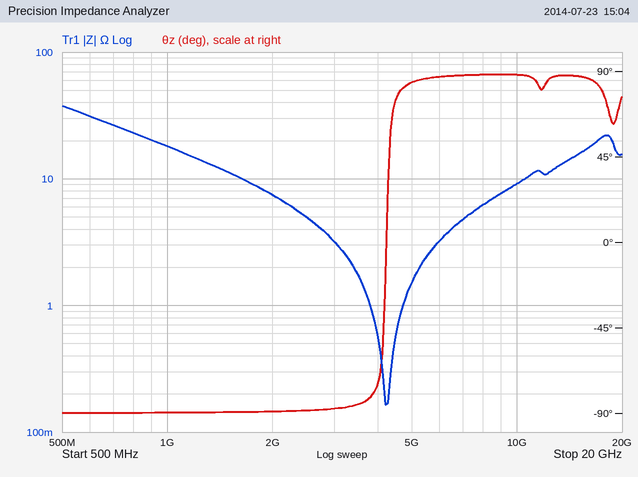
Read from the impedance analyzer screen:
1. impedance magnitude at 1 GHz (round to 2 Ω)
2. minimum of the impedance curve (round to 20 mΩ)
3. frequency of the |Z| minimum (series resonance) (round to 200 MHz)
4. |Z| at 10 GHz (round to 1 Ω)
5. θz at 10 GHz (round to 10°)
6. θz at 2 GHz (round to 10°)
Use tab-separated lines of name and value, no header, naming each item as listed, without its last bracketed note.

impedance magnitude at 1 GHz	18 Ω
minimum of the impedance curve	160 mΩ
frequency of the |Z| minimum (series resonance)	4.2 GHz
|Z| at 10 GHz	9 Ω
θz at 10 GHz	90°
θz at 2 GHz	-90°
